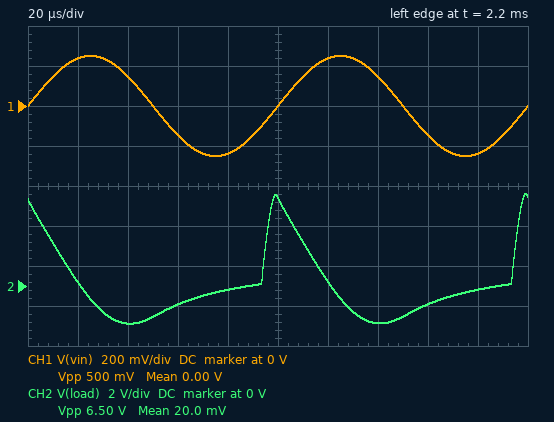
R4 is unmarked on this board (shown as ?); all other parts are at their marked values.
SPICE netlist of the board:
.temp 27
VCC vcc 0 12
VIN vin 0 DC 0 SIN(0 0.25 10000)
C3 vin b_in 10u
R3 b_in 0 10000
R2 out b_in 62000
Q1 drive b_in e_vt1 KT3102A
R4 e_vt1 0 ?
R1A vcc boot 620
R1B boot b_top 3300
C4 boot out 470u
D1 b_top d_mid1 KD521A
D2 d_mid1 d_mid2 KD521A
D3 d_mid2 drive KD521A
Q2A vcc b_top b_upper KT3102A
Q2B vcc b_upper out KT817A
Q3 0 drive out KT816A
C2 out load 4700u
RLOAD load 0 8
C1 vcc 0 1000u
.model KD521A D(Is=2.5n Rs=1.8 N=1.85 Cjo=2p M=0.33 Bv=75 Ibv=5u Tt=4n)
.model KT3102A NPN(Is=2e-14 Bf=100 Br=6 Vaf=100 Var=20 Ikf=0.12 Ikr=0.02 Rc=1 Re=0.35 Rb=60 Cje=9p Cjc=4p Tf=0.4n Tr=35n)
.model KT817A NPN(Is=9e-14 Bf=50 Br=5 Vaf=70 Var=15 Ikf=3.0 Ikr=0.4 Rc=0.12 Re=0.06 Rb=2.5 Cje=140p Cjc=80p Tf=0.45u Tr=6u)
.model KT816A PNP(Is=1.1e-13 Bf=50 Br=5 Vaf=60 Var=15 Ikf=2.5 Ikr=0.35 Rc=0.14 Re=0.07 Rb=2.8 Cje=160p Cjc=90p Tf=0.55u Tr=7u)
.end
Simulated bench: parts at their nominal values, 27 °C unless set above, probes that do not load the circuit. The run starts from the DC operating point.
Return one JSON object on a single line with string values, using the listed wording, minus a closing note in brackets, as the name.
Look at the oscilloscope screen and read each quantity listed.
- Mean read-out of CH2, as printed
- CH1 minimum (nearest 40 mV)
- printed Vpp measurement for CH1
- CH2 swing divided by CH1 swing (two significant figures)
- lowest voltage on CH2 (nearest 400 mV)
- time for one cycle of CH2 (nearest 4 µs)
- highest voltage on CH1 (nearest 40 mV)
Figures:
{"Mean read-out of CH2, as printed": "20.0 mV", "CH1 minimum": "-240 mV", "printed Vpp measurement for CH1": "500 mV", "CH2 swing divided by CH1 swing": "13", "lowest voltage on CH2": "-2.0 V", "time for one cycle of CH2": "100 µs", "highest voltage on CH1": "240 mV"}
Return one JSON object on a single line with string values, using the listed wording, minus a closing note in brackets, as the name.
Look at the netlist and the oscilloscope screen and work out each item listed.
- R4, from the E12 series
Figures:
{"R4, from the E12 series": "15 Ω"}
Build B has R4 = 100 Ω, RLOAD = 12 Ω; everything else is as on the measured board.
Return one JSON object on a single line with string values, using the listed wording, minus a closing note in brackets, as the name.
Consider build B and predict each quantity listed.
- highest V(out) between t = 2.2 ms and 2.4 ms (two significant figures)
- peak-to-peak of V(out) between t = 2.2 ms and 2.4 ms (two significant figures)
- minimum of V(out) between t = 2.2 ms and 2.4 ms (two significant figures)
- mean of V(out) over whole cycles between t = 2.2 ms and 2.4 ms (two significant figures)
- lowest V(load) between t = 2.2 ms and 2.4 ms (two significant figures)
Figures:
{"highest V(out) between t = 2.2 ms and 2.4 ms": "11 V", "peak-to-peak of V(out) between t = 2.2 ms and 2.4 ms": "5.1 V", "minimum of V(out) between t = 2.2 ms and 2.4 ms": "6.1 V", "mean of V(out) over whole cycles between t = 2.2 ms and 2.4 ms": "8.0 V", "lowest V(load) between t = 2.2 ms and 2.4 ms": "-340 mV"}
